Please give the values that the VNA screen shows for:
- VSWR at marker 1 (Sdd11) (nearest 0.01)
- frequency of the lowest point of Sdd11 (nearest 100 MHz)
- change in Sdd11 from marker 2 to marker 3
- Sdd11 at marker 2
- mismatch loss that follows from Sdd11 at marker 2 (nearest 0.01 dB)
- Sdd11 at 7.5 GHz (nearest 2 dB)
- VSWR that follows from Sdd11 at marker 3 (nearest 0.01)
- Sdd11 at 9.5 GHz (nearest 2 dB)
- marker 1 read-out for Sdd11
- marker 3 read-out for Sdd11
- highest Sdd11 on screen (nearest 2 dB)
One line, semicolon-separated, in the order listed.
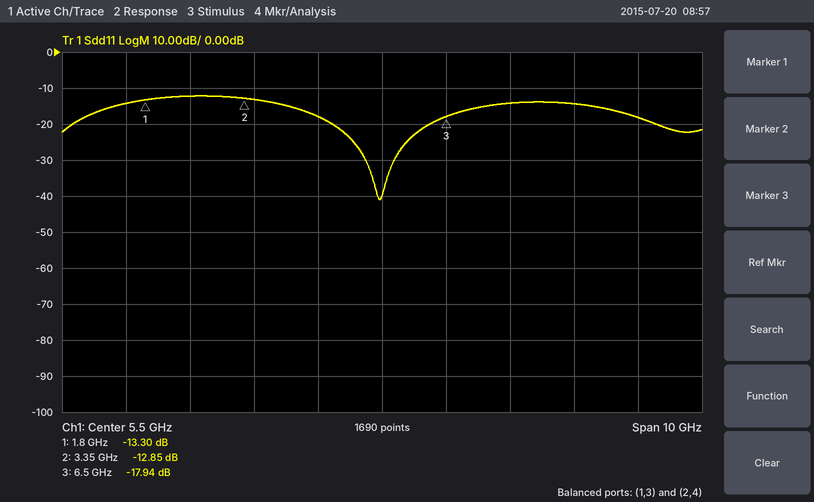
1.55; 5.5 GHz; -5.09 dB; -12.85 dB; 0.23 dB; -14 dB; 1.29; -18 dB; -13.30 dB; -17.94 dB; -12 dB
